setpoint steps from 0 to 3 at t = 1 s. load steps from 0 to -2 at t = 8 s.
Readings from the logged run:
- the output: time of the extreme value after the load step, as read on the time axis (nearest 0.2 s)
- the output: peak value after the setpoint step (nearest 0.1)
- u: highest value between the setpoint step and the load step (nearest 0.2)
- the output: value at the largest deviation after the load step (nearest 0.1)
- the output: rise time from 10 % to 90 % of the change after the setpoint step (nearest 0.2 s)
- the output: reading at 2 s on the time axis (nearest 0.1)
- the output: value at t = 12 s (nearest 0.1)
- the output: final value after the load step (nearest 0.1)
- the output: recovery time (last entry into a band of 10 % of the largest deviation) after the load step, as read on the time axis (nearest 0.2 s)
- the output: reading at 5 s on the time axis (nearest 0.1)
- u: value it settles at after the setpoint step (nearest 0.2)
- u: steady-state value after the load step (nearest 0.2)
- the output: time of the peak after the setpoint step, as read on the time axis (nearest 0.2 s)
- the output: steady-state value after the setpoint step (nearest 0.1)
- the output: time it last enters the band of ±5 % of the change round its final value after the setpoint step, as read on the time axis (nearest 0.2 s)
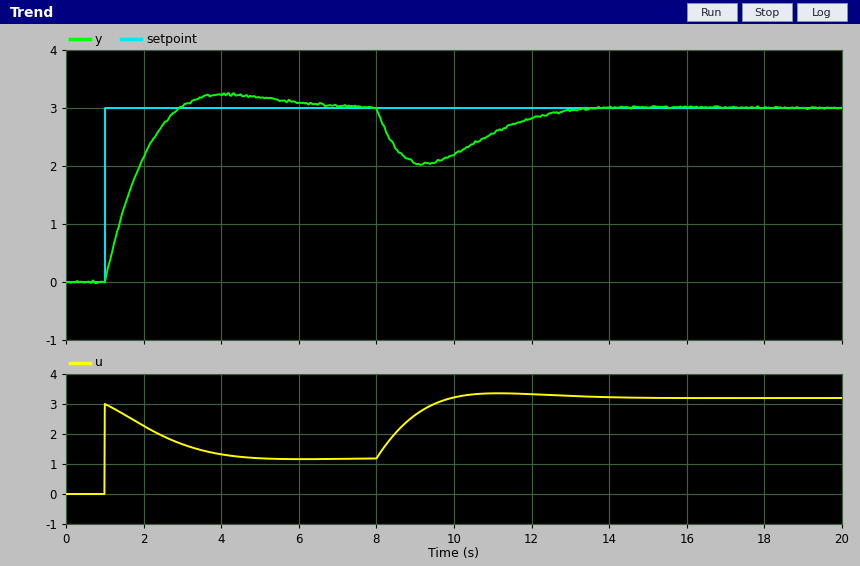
9.2 s
3.2
3.0
2.0
1.4 s
2.2
2.8
3.0
12.4 s
3.2
1.2
3.2
4.2 s
3.0
5.4 s
